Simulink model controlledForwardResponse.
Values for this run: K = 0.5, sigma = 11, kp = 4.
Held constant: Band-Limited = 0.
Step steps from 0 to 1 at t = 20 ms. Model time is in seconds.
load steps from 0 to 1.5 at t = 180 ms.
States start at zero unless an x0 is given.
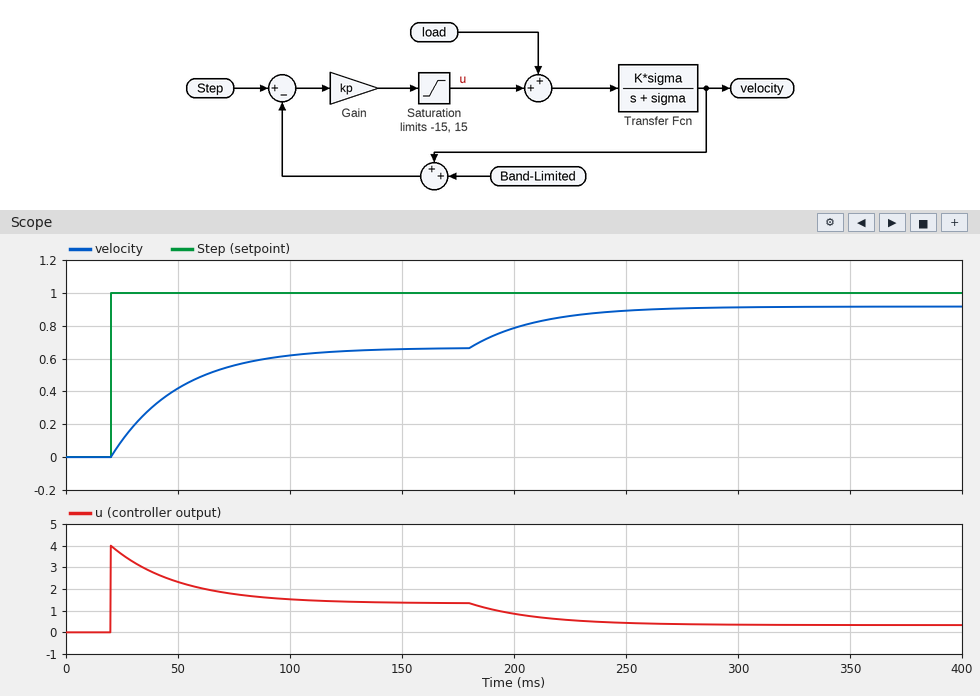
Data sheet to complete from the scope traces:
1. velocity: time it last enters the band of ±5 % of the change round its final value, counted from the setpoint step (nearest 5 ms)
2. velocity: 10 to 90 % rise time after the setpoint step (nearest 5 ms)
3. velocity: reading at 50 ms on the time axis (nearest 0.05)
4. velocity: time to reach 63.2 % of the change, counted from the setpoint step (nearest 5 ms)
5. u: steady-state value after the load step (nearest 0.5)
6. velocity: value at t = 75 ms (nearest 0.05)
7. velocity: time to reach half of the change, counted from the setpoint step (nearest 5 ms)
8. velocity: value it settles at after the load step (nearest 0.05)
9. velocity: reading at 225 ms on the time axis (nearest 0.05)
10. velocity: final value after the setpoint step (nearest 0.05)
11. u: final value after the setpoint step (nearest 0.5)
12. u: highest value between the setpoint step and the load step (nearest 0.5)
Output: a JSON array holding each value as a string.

["90 ms", "65 ms", "0.40", "30 ms", "0.5", "0.55", "20 ms", "0.90", "0.85", "0.65", "1.5", "4.0"]
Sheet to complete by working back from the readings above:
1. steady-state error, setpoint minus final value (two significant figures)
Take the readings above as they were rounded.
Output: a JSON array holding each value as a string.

["0.35"]
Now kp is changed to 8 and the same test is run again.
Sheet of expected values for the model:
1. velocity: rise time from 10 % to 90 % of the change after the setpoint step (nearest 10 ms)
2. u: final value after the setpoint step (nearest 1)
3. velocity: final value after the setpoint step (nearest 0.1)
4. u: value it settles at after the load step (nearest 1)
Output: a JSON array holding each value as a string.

["40 ms", "2", "0.8", "0"]
